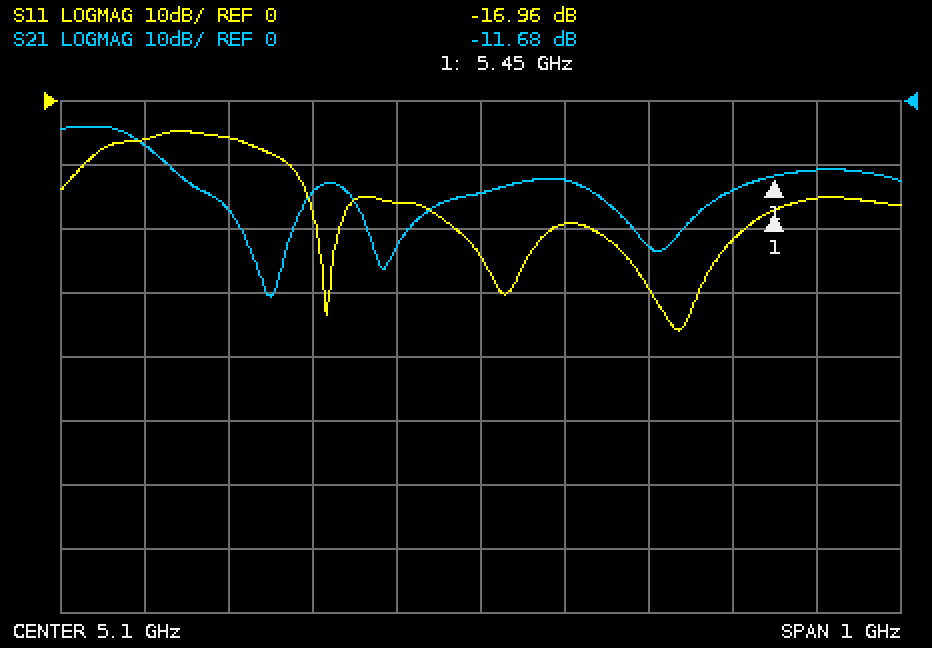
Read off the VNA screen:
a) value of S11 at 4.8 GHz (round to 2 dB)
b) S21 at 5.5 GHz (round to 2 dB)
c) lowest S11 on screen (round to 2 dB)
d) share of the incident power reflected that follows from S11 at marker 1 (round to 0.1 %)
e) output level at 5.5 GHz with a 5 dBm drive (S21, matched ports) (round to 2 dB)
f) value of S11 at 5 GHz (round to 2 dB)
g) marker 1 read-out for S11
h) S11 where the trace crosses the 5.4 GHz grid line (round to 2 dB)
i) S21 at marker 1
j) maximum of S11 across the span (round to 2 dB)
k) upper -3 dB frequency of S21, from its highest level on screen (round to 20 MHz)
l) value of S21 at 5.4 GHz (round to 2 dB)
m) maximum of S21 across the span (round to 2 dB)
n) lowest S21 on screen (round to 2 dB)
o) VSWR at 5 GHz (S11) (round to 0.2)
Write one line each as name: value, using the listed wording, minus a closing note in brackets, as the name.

value of S11 at 4.8 GHz: -6 dB
S21 at 5.5 GHz: -10 dB
lowest S11 on screen: -36 dB
share of the incident power reflected that follows from S11 at marker 1: 2.0 %
output level at 5.5 GHz with a 5 dBm drive (S21, matched ports): -6 dBm
value of S11 at 5 GHz: -16 dB
marker 1 read-out for S11: -16.96 dB
S11 where the trace crosses the 5.4 GHz grid line: -22 dB
S21 at marker 1: -11.68 dB
maximum of S11 across the span: -4 dB
upper -3 dB frequency of S21, from its highest level on screen: 4.70 GHz
value of S21 at 5.4 GHz: -14 dB
maximum of S21 across the span: -4 dB
lowest S21 on screen: -30 dB
VSWR at 5 GHz (S11): 1.4
